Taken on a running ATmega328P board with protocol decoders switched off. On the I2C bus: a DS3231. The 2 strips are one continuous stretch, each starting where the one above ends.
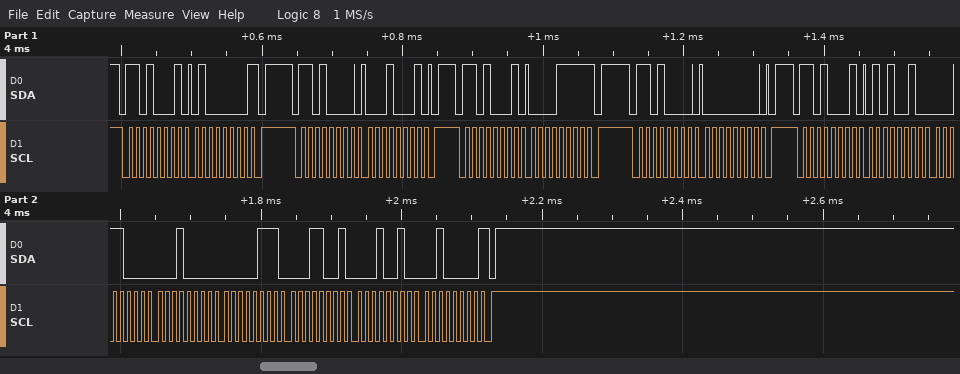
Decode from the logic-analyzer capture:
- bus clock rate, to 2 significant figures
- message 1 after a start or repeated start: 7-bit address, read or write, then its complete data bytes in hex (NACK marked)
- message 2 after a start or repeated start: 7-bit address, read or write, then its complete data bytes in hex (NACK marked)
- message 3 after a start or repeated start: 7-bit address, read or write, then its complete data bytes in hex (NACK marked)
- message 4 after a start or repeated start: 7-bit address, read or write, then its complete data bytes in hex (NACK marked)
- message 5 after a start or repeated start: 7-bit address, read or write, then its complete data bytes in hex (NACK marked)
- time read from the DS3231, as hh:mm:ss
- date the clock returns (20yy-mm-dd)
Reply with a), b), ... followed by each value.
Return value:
a) 100 kHz
b) 0x68 read: 40 NACK
c) 0x68 write: 11
d) 0x68 read: 0F NACK
e) 0x68 write: 00
f) 0x68 read: 52 18 10 07 19 12 20 NACK
g) 10:18:52
h) 2020-12-19
